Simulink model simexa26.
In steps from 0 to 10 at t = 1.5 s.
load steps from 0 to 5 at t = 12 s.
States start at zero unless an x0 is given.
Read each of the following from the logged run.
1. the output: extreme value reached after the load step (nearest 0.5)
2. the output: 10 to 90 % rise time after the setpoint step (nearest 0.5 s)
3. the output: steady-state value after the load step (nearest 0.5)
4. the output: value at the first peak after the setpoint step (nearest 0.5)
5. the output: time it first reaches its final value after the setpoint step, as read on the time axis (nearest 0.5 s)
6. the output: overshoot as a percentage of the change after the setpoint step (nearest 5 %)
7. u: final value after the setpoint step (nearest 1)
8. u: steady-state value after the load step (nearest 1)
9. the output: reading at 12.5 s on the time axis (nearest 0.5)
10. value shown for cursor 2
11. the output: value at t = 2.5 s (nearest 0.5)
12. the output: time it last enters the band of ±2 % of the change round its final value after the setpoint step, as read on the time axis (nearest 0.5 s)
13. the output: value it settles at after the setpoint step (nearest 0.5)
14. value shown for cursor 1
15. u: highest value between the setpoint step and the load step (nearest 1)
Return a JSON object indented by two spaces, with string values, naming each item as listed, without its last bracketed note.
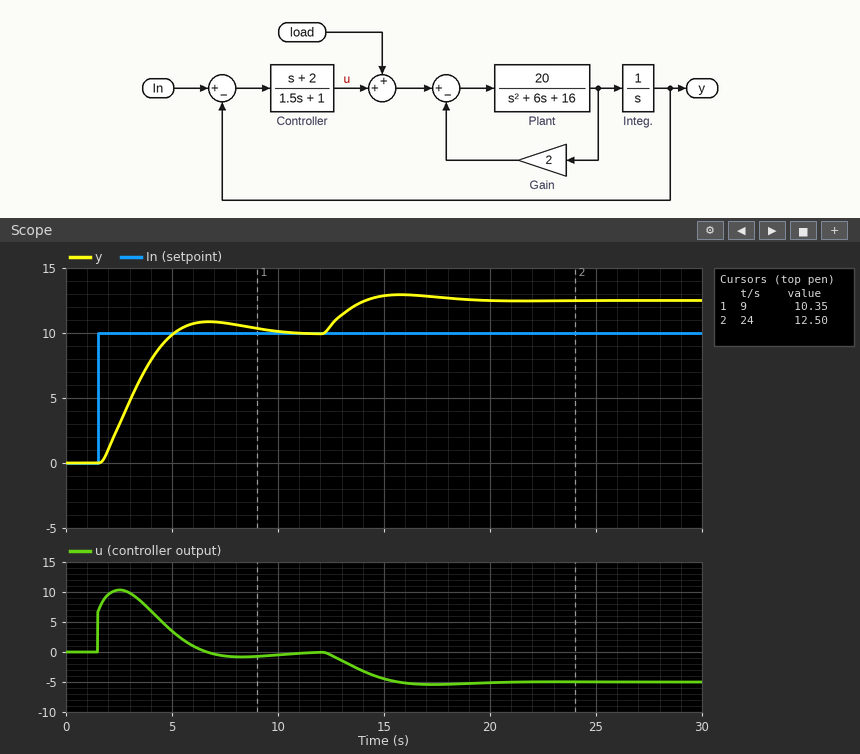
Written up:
{
  "the output: extreme value reached after the load step": "13.0",
  "the output: 10 to 90 % rise time after the setpoint step": "2.5 s",
  "the output: steady-state value after the load step": "12.5",
  "the output: value at the first peak after the setpoint step": "11.0",
  "the output: time it first reaches its final value after the setpoint step, as read on the time axis": "5.0 s",
  "the output: overshoot as a percentage of the change after the setpoint step": "10 %",
  "u: final value after the setpoint step": "0",
  "u: steady-state value after the load step": "-5",
  "the output: reading at 12.5 s on the time axis": "10.5",
  "value shown for cursor 2": "12.50",
  "the output: value at t = 2.5 s": "3.0",
  "the output: time it last enters the band of ±2 % of the change round its final value after the setpoint step, as read on the time axis": "9.5 s",
  "the output: value it settles at after the setpoint step": "10.0",
  "value shown for cursor 1": "10.35",
  "u: highest value between the setpoint step and the load step": "10"
}
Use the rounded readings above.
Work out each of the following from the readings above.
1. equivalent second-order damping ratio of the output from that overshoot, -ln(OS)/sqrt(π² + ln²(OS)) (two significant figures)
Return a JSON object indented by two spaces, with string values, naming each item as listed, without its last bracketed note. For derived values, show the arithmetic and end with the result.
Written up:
{
  "equivalent second-order damping ratio of the output from that overshoot, -ln(OS)/sqrt(π² + ln²(OS))": "ln(0.1) = -2.303; 2.303 / sqrt(9.870 + 5.302) = 0.59"
}
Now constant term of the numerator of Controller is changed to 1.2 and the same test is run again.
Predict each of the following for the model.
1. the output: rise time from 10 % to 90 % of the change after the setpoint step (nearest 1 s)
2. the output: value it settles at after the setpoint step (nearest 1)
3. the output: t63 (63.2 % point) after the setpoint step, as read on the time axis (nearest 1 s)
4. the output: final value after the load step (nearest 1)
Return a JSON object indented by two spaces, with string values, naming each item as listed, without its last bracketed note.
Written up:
{
  "the output: rise time from 10 % to 90 % of the change after the setpoint step": "4 s",
  "the output: value it settles at after the setpoint step": "10",
  "the output: t63 (63.2 % point) after the setpoint step, as read on the time axis": "4 s",
  "the output: final value after the load step": "14"
}
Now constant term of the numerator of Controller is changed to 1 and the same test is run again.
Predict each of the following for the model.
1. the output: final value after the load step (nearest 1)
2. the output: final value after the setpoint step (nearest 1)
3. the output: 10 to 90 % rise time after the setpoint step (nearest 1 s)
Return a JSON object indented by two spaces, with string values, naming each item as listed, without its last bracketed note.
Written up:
{
  "the output: final value after the load step": "15",
  "the output: final value after the setpoint step": "10",
  "the output: 10 to 90 % rise time after the setpoint step": "5 s"
}
